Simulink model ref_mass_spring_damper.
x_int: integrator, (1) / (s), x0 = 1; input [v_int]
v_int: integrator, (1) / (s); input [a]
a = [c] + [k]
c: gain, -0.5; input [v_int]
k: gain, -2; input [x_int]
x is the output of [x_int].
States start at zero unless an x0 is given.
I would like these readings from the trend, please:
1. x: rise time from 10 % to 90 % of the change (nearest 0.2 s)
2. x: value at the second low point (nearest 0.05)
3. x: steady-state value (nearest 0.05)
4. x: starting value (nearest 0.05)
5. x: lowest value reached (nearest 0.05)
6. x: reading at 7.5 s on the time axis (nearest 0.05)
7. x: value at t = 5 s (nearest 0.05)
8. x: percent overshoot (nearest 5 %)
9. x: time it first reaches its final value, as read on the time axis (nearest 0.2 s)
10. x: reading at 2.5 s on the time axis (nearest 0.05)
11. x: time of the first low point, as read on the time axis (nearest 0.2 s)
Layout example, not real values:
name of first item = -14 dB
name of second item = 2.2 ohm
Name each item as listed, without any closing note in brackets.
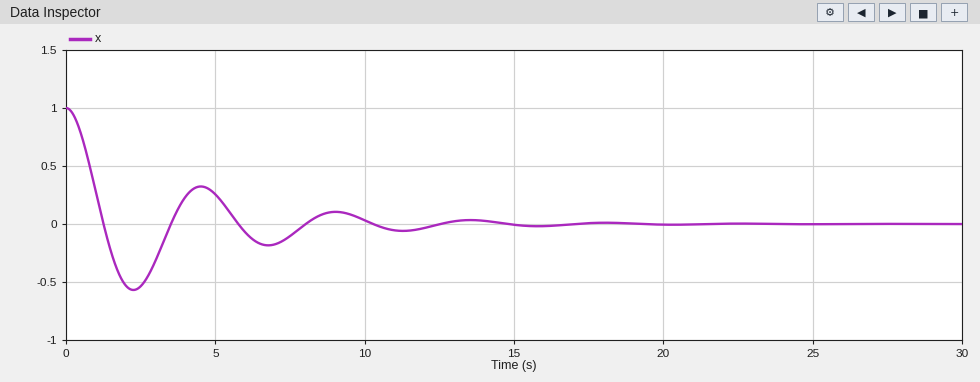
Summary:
x: rise time from 10 % to 90 % of the change = 0.8 s
x: value at the second low point = -0.20
x: steady-state value = 0.00
x: starting value = 1.00
x: lowest value reached = -0.55
x: reading at 7.5 s on the time axis = -0.10
x: value at t = 5 s = 0.25
x: percent overshoot = 55 %
x: time it first reaches its final value, as read on the time axis = 1.2 s
x: reading at 2.5 s on the time axis = -0.55
x: time of the first low point, as read on the time axis = 2.2 s
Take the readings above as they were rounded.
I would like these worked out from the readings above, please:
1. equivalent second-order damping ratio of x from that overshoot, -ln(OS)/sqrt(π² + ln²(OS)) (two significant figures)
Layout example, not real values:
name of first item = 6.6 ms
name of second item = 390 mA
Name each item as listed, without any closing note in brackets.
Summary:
equivalent second-order damping ratio of x from that overshoot, -ln(OS)/sqrt(π² + ln²(OS)) = 0.19
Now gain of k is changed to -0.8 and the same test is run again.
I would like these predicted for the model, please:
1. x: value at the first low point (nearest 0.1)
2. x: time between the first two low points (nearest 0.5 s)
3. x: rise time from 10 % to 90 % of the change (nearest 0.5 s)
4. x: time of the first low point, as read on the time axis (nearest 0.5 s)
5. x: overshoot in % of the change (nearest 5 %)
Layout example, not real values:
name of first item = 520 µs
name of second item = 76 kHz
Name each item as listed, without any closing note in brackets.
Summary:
x: value at the first low point = -0.4
x: time between the first two low points = 7.5 s
x: rise time from 10 % to 90 % of the change = 1.5 s
x: time of the first low point, as read on the time axis = 3.5 s
x: overshoot in % of the change = 40 %
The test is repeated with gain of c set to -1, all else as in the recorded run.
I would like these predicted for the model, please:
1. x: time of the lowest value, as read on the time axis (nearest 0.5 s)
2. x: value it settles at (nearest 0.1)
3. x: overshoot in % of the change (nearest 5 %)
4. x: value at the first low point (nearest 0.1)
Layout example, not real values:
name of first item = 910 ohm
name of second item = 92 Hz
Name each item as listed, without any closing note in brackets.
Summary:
x: time of the lowest value, as read on the time axis = 2.5 s
x: value it settles at = 0.0
x: overshoot in % of the change = 30 %
x: value at the first low point = -0.3
